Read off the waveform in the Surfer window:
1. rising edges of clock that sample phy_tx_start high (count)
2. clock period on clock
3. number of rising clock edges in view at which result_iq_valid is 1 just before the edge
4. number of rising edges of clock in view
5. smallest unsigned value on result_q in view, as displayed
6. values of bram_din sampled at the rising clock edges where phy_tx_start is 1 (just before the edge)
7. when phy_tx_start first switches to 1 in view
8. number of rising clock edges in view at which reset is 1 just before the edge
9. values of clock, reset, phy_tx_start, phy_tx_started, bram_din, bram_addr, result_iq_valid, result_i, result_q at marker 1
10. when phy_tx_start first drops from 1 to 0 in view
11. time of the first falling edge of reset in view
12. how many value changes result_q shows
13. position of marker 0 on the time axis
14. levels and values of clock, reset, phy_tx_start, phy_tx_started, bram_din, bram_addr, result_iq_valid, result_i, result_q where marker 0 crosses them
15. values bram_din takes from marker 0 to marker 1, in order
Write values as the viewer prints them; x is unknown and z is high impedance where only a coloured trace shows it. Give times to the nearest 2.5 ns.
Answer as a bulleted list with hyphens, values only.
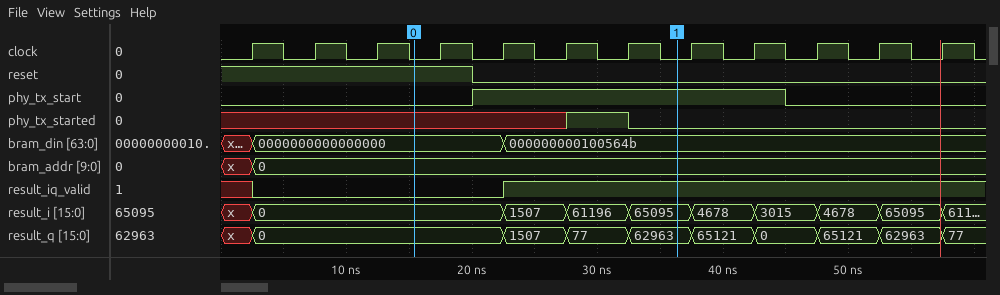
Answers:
- 5
- 5 ns
- 7
- 12
- 0
- 0000000000000000, 000000000100564b, 000000000100564b, 000000000100564b, 000000000100564b
- 20 ns
- 4
- clock=0, reset=0, phy_tx_start=1, phy_tx_started=0, bram_din=000000000100564b, bram_addr=0, result_iq_valid=1, result_i=65095, result_q=62963
- 45 ns
- 20 ns
- 9
- 15 ns
- clock=0, reset=1, phy_tx_start=0, phy_tx_started=x, bram_din=0000000000000000, bram_addr=0, result_iq_valid=0, result_i=0, result_q=0
- 0000000000000000, 000000000100564b
